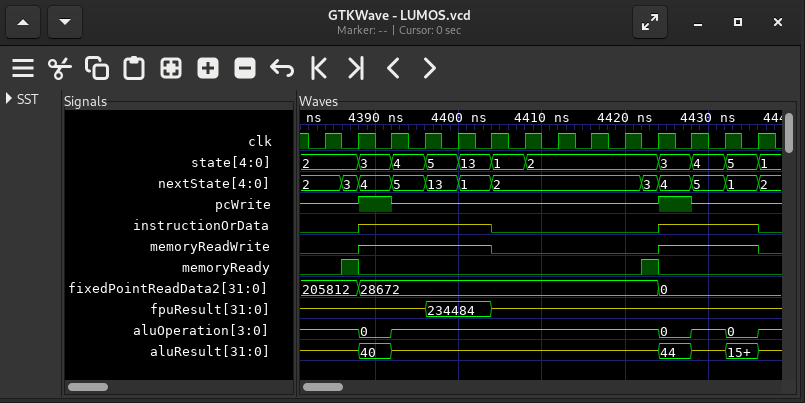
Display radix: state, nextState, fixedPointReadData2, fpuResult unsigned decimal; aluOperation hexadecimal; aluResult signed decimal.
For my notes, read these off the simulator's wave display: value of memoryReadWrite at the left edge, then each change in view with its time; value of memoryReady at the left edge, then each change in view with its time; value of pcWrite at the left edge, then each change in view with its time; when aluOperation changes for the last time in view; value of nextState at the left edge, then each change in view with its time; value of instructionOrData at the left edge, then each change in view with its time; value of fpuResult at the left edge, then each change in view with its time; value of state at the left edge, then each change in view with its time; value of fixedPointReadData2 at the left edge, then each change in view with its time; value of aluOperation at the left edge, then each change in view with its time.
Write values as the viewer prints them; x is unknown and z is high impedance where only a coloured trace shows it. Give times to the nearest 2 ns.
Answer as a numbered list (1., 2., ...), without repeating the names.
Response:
1. 0, z at 4388 ns, 0 at 4404 ns, z at 4424 ns, 0 at 4436 ns
2. 0, 1 at 4386 ns, 0 at 4388 ns, 1 at 4422 ns, 0 at 4424 ns
3. z, 1 at 4388 ns, z at 4392 ns, 1 at 4424 ns, z at 4428 ns
4. 4436 ns
5. 2, 3 at 4386 ns, 4 at 4388 ns, 5 at 4392 ns, 13 at 4396 ns, 1 at 4400 ns, 2 at 4404 ns, 3 at 4422 ns, 4 at 4424 ns, 5 at 4428 ns, 1 at 4432 ns, 2 at 4436 ns
6. 0, z at 4388 ns, 0 at 4404 ns, z at 4424 ns, 0 at 4436 ns
7. z, 234484 at 4396 ns, z at 4404 ns
8. 2, 3 at 4388 ns, 4 at 4392 ns, 5 at 4396 ns, 13 at 4400 ns, 1 at 4404 ns, 2 at 4408 ns, 3 at 4424 ns, 4 at 4428 ns, 5 at 4432 ns, 1 at 4436 ns
9. 205812, 28672 at 4388 ns, 0 at 4424 ns
10. z, 0 at 4388 ns, z at 4392 ns, 0 at 4424 ns, z at 4428 ns, 0 at 4432 ns, z at 4436 ns
